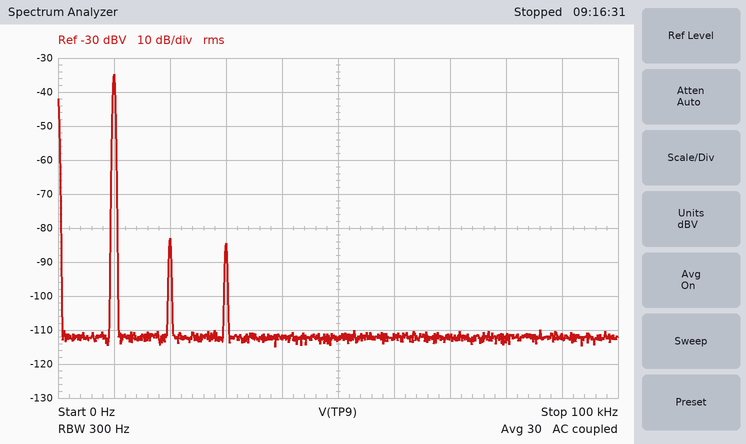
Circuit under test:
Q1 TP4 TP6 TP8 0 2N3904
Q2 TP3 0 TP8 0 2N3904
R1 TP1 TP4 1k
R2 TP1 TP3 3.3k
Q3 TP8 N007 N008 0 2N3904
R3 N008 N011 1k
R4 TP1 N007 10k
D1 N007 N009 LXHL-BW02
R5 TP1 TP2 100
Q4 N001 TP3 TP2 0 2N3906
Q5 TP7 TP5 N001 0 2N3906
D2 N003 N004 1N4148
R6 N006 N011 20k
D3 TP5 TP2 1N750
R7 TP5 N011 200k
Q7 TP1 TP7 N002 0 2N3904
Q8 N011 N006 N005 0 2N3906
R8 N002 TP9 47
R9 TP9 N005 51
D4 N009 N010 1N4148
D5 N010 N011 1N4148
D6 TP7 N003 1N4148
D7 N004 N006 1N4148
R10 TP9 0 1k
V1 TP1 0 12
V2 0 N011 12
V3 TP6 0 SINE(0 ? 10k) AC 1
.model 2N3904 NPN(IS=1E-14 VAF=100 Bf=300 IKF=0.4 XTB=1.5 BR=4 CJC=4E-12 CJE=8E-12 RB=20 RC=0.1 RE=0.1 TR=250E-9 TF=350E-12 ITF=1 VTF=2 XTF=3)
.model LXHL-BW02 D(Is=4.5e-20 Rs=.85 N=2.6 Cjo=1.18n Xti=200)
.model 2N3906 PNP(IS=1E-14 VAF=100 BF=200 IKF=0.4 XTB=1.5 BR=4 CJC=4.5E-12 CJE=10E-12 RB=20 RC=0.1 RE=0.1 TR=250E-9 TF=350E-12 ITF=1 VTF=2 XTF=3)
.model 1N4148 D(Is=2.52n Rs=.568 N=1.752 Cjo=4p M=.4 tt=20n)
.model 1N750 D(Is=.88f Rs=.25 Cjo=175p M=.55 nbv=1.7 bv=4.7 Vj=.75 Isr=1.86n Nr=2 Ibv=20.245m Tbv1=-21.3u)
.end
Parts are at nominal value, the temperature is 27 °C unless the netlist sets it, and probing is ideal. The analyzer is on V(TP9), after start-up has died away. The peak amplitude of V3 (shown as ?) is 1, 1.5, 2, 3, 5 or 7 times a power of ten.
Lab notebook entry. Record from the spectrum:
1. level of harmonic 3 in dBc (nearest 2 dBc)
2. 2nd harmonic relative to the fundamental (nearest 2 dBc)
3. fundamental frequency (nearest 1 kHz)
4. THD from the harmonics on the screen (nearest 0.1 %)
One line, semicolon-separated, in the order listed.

-50 dBc; -48 dBc; 10 kHz; 0.5 %
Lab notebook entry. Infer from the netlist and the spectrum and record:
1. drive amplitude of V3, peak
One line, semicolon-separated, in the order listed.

10 mV
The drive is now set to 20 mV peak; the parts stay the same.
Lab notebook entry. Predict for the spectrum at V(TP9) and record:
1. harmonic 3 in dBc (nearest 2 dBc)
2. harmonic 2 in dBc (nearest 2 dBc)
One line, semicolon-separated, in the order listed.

-38 dBc; -42 dBc
